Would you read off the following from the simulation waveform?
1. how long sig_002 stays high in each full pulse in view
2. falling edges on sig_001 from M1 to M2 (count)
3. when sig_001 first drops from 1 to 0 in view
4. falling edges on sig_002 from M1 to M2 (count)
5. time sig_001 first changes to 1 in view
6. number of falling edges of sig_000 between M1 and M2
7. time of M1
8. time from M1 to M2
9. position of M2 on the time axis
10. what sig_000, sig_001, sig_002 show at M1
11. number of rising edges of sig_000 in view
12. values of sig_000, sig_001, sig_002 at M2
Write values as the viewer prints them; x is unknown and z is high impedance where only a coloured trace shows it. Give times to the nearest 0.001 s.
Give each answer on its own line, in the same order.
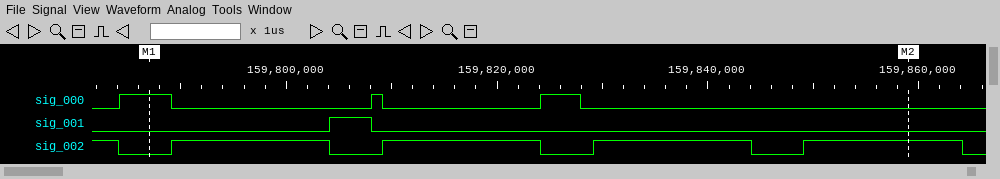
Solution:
0.015 s, 0.015 s, 0.015 s, 0.015 s
1
159.808 s
3
159.804 s
3
159.787 s
0.072 s
159.859 s
sig_000=1, sig_001=0, sig_002=0
3
sig_000=0, sig_001=0, sig_002=1
